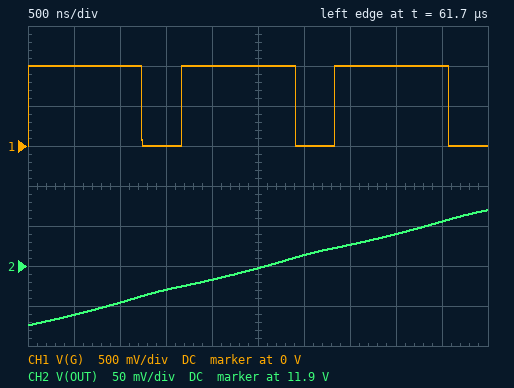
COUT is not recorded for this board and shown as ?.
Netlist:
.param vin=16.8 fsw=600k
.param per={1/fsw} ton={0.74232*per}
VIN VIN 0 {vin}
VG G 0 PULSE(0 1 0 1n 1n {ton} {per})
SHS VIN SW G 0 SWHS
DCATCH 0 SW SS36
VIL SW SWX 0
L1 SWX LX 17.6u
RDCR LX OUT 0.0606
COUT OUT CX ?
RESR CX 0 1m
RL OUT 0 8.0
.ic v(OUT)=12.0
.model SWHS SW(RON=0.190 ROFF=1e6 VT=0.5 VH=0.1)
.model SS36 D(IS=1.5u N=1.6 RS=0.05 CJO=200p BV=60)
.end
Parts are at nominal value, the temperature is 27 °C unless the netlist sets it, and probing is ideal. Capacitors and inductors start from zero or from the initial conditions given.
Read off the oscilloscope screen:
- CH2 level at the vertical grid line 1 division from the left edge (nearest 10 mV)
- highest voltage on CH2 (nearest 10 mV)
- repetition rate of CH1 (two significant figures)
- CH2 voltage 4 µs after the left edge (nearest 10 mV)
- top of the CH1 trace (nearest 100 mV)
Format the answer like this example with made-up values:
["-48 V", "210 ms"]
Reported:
["11.84 V", "11.97 V", "600 kHz", "11.94 V", "1.0 V"]
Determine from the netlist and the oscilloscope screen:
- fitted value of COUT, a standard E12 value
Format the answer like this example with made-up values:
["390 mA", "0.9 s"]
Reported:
["27 µF"]
